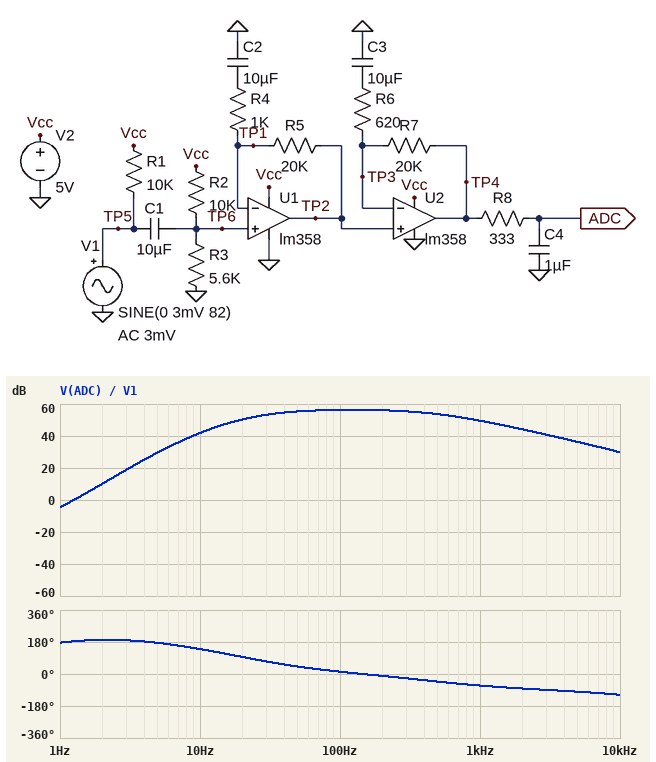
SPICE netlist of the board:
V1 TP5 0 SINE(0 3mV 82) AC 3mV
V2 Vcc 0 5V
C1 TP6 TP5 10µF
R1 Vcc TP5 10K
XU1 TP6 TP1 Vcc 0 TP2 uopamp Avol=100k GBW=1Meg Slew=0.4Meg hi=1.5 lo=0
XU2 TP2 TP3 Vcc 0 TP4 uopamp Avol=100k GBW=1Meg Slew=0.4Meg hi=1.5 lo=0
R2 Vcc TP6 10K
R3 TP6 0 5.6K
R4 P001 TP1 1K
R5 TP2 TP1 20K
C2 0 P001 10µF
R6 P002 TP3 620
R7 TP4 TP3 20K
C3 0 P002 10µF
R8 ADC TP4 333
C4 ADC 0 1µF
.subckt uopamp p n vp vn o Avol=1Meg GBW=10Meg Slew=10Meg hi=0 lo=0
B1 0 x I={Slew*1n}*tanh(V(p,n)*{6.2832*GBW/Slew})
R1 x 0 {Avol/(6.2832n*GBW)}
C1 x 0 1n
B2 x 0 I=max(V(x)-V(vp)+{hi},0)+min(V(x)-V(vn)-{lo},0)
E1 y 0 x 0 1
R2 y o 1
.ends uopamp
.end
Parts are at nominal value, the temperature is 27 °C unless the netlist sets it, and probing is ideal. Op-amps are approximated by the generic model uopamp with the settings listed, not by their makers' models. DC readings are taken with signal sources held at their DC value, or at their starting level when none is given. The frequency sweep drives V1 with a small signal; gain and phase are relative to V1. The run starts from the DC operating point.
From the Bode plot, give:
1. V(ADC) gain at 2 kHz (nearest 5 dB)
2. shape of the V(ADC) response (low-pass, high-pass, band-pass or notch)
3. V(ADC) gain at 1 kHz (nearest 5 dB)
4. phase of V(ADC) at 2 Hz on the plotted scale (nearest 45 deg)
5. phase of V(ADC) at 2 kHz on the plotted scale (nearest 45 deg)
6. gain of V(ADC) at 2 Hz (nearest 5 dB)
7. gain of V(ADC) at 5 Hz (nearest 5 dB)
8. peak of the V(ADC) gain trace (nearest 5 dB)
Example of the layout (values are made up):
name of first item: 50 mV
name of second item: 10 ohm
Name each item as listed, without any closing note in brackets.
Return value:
V(ADC) gain at 2 kHz: 45 dB
shape of the V(ADC) response: band-pass
V(ADC) gain at 1 kHz: 50 dB
phase of V(ADC) at 2 Hz on the plotted scale: 180 deg
phase of V(ADC) at 2 kHz on the plotted scale: -90 deg
gain of V(ADC) at 2 Hz: 10 dB
gain of V(ADC) at 5 Hz: 30 dB
peak of the V(ADC) gain trace: 55 dB
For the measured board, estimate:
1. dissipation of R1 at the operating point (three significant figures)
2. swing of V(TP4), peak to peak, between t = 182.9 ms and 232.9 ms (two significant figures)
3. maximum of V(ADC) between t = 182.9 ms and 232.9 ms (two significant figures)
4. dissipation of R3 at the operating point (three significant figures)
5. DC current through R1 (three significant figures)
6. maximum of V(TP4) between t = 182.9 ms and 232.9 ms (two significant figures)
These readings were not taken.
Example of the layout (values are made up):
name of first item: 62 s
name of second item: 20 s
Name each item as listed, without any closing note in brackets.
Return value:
dissipation of R1 at the operating point: 2.50 mW
swing of V(TP4), peak to peak, between t = 182.9 ms and 232.9 ms: 3.5 V
maximum of V(ADC) between t = 182.9 ms and 232.9 ms: 3.5 V
dissipation of R3 at the operating point: 575 µW
DC current through R1: 500 µA
maximum of V(TP4) between t = 182.9 ms and 232.9 ms: 3.5 V
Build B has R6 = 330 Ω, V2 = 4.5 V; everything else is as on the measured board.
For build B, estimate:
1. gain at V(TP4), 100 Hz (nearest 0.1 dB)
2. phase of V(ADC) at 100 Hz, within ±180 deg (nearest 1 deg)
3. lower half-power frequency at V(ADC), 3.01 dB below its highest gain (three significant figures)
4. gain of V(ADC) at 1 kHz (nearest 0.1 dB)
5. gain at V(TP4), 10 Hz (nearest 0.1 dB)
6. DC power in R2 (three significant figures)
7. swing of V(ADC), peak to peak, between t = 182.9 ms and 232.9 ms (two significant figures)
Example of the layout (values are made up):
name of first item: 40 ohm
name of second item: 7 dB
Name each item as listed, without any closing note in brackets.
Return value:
gain at V(TP4), 100 Hz: 61.2 dB
phase of V(ADC) at 100 Hz, within ±180 deg: 24 deg
lower half-power frequency at V(ADC), 3.01 dB below its highest gain: 45.2 Hz
gain of V(ADC) at 1 kHz: 54.9 dB
gain at V(TP4), 10 Hz: 42.2 dB
DC power in R2: 832 µW
swing of V(ADC), peak to peak, between t = 182.9 ms and 232.9 ms: 3.0 V
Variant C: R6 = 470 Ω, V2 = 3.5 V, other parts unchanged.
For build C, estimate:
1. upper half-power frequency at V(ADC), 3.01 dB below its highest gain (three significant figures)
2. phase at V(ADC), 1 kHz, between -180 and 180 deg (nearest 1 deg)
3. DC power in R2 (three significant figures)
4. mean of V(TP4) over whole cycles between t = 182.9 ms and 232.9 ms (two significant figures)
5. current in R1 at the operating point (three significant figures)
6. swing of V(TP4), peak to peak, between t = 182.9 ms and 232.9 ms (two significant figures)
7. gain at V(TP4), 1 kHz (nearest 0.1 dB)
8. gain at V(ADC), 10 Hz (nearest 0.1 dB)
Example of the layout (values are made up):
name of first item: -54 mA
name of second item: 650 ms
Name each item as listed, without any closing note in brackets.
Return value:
upper half-power frequency at V(ADC), 3.01 dB below its highest gain: 549 Hz
phase at V(ADC), 1 kHz, between -180 and 180 deg: -65 deg
DC power in R2: 503 µW
mean of V(TP4) over whole cycles between t = 182.9 ms and 232.9 ms: 1.2 V
current in R1 at the operating point: 350 µA
swing of V(TP4), peak to peak, between t = 182.9 ms and 232.9 ms: 2.0 V
gain at V(TP4), 1 kHz: 59.2 dB
gain at V(ADC), 10 Hz: 42.1 dB
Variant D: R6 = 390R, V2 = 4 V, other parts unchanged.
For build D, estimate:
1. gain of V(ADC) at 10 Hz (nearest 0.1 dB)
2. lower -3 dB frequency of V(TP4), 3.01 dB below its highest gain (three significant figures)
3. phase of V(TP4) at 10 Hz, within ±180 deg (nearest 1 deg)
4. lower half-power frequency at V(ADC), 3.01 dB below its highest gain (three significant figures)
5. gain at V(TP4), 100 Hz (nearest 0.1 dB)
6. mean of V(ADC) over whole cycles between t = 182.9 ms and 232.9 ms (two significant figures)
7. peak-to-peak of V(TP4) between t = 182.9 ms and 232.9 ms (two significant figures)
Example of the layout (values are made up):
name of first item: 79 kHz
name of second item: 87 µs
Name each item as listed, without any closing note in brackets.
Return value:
gain of V(ADC) at 10 Hz: 42.1 dB
lower -3 dB frequency of V(TP4), 3.01 dB below its highest gain: 46.2 Hz
phase of V(TP4) at 10 Hz, within ±180 deg: 149 deg
lower half-power frequency at V(ADC), 3.01 dB below its highest gain: 40.3 Hz
gain at V(TP4), 100 Hz: 60.0 dB
mean of V(ADC) over whole cycles between t = 182.9 ms and 232.9 ms: 1.4 V
peak-to-peak of V(TP4) between t = 182.9 ms and 232.9 ms: 2.5 V
